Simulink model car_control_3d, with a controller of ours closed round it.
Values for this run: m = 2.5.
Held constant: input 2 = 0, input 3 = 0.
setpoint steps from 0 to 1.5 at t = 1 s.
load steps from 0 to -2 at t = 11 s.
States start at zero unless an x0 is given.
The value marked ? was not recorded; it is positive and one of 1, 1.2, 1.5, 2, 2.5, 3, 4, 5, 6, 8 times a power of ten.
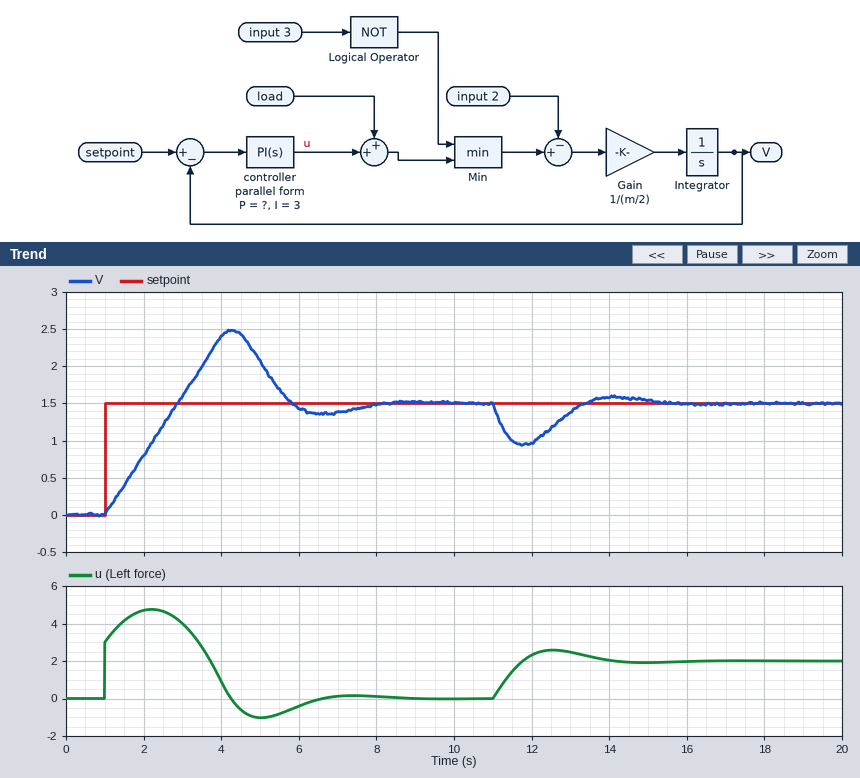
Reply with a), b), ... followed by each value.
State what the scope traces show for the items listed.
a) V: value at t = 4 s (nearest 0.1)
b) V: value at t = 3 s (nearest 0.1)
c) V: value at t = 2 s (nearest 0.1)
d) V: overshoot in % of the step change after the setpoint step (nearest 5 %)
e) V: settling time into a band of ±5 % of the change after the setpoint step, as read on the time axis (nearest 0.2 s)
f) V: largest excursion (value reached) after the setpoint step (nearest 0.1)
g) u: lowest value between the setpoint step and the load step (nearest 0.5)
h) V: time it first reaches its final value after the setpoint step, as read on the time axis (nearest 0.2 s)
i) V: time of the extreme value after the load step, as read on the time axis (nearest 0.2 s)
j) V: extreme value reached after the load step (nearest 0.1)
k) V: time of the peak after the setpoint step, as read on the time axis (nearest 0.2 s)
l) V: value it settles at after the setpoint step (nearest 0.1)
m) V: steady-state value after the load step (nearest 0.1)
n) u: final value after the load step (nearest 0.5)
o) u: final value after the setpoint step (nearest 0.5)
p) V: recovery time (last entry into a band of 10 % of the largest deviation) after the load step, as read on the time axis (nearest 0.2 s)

a) 2.4
b) 1.6
c) 0.8
d) 65 %
e) 7.4 s
f) 2.5
g) -1.0
h) 2.8 s
i) 11.8 s
j) 0.9
k) 4.2 s
l) 1.5
m) 1.5
n) 2.0
o) 0.0
p) 14.8 s
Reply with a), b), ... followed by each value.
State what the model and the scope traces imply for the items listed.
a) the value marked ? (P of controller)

a) 2
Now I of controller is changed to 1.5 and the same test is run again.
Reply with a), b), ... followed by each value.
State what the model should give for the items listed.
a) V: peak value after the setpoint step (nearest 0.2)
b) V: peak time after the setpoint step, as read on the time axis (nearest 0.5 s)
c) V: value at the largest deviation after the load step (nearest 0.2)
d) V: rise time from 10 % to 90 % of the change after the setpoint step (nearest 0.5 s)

a) 2.2
b) 4.0 s
c) 0.8
d) 1.5 s
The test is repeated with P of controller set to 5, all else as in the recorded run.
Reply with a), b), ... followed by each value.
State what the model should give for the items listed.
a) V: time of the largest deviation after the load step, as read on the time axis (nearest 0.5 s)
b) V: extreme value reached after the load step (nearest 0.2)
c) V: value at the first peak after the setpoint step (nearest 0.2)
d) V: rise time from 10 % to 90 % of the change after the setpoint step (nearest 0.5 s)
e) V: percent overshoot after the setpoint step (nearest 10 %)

a) 11.5 s
b) 1.2
c) 2.2
d) 1.5 s
e) 40 %
